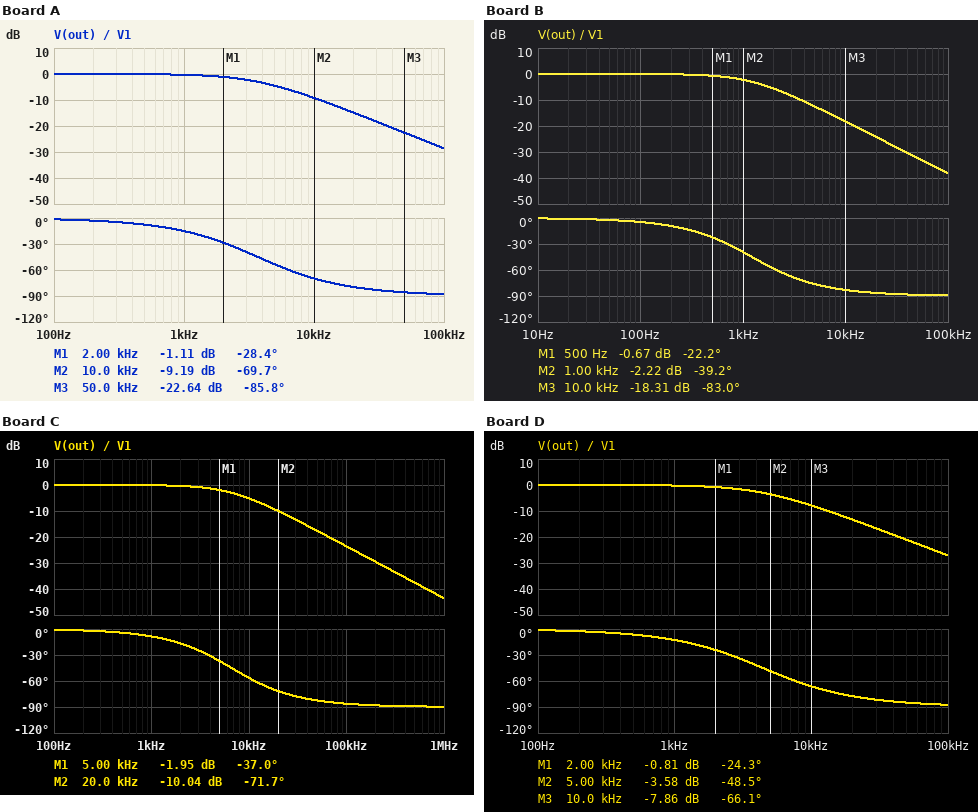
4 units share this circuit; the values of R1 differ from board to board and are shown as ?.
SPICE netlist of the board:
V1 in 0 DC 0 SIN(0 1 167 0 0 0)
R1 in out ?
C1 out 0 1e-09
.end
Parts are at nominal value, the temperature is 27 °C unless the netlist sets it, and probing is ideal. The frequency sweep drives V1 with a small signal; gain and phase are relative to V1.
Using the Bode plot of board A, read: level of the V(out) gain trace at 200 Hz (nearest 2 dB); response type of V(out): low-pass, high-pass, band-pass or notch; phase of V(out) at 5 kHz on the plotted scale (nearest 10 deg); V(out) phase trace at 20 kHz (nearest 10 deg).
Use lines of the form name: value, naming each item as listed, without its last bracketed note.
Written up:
level of the V(out) gain trace at 200 Hz: 0 dB
response type of V(out): low-pass, high-pass, band-pass or notch: low-pass
phase of V(out) at 5 kHz on the plotted scale: -50 deg
V(out) phase trace at 20 kHz: -80 deg
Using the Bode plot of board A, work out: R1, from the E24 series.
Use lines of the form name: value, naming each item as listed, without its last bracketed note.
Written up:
R1, from the E24 series: 43 kΩ
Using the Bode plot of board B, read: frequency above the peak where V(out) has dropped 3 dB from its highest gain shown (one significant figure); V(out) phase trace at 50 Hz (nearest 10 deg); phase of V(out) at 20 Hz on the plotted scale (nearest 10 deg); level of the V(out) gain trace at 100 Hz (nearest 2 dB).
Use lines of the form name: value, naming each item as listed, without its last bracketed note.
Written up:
frequency above the peak where V(out) has dropped 3 dB from its highest gain shown: 1 kHz
V(out) phase trace at 50 Hz: 0 deg
phase of V(out) at 20 Hz on the plotted scale: 0 deg
level of the V(out) gain trace at 100 Hz: 0 dB
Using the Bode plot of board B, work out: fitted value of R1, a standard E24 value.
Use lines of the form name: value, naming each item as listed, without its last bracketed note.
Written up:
fitted value of R1, a standard E24 value: 130 kΩ
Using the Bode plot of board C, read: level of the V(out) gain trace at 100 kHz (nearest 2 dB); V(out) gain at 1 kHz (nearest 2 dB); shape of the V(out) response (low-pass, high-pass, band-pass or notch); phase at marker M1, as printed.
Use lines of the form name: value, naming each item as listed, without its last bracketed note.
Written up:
level of the V(out) gain trace at 100 kHz: -24 dB
V(out) gain at 1 kHz: 0 dB
shape of the V(out) response: low-pass
phase at marker M1, as printed: -37.0 deg
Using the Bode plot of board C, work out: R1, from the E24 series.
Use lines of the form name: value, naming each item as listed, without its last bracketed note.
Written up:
R1, from the E24 series: 24 kΩ
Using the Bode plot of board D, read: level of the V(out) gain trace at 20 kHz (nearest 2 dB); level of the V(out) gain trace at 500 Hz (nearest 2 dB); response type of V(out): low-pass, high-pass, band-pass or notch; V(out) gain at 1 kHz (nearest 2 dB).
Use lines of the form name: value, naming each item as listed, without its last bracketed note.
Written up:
level of the V(out) gain trace at 20 kHz: -14 dB
level of the V(out) gain trace at 500 Hz: 0 dB
response type of V(out): low-pass, high-pass, band-pass or notch: low-pass
V(out) gain at 1 kHz: 0 dB
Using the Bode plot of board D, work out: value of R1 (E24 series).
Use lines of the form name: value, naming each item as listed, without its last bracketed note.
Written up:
value of R1: 36 kΩ
